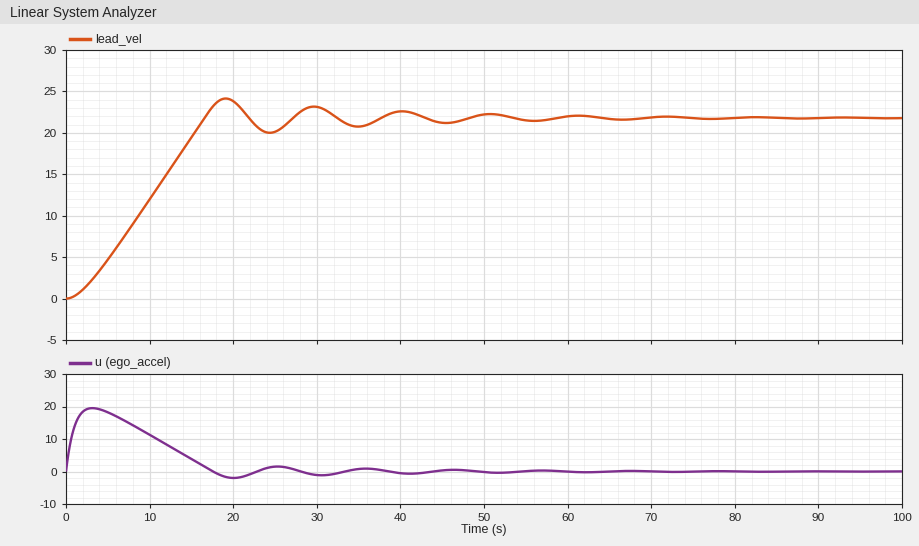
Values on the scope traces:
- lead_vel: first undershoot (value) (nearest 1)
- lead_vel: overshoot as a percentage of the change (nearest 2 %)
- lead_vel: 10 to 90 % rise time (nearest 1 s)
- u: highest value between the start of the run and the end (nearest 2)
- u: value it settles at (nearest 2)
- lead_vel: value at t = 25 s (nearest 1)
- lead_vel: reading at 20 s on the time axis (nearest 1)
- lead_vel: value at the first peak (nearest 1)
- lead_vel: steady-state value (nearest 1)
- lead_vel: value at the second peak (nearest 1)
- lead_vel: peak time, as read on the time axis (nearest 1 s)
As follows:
20
10 %
12 s
20
0
20
24
24
22
23
19 s
